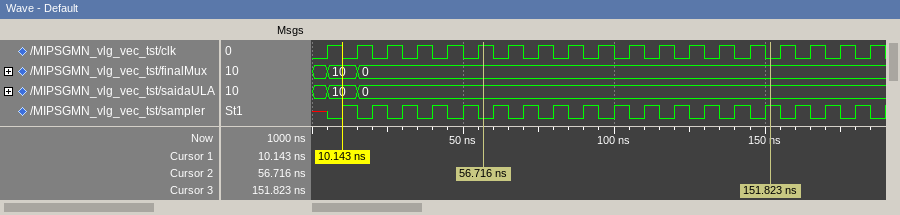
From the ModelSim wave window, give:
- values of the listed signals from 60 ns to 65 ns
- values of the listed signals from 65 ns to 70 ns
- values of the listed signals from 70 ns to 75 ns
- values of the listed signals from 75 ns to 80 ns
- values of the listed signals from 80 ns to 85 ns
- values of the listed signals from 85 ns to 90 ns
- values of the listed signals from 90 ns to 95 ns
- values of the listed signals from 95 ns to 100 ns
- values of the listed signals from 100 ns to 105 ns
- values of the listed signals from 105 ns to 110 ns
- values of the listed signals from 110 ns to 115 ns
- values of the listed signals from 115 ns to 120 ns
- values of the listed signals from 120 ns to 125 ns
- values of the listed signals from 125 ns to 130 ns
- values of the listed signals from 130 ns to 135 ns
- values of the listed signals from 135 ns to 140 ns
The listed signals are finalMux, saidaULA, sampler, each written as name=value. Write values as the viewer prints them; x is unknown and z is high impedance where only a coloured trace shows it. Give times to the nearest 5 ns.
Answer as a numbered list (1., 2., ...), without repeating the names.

1. finalMux=0, saidaULA=0, sampler=1
2. finalMux=0, saidaULA=0, sampler=0
3. finalMux=0, saidaULA=0, sampler=1
4. finalMux=0, saidaULA=0, sampler=0
5. finalMux=0, saidaULA=0, sampler=1
6. finalMux=0, saidaULA=0, sampler=0
7. finalMux=0, saidaULA=0, sampler=1
8. finalMux=0, saidaULA=0, sampler=0
9. finalMux=0, saidaULA=0, sampler=1
10. finalMux=0, saidaULA=0, sampler=0
11. finalMux=0, saidaULA=0, sampler=1
12. finalMux=0, saidaULA=0, sampler=0
13. finalMux=0, saidaULA=0, sampler=1
14. finalMux=0, saidaULA=0, sampler=0
15. finalMux=0, saidaULA=0, sampler=1
16. finalMux=0, saidaULA=0, sampler=0
